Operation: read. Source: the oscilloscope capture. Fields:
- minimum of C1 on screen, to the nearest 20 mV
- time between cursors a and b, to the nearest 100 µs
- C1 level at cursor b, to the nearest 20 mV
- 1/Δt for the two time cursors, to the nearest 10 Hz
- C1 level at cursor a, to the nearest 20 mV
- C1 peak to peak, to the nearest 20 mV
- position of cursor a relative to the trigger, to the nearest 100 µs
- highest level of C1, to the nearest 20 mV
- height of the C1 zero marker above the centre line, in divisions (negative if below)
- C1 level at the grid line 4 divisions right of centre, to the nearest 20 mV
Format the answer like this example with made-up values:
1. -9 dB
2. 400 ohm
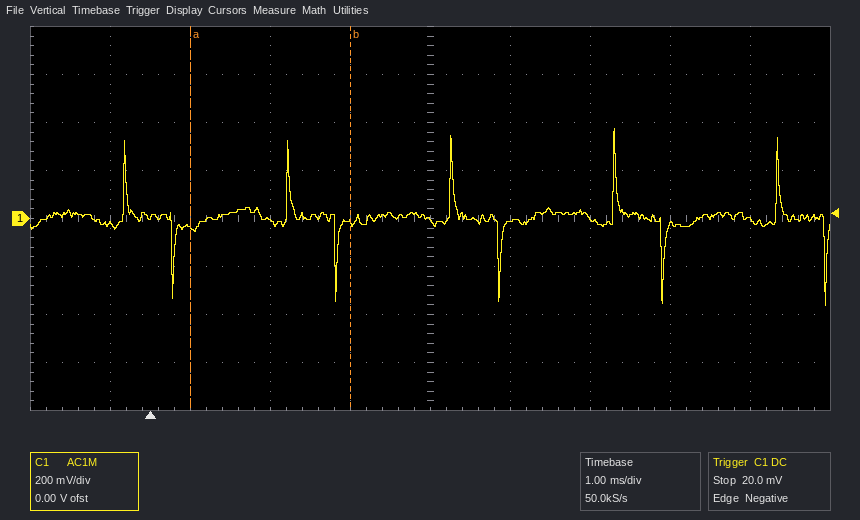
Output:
1. -360 mV
2. 2.0 ms
3. -20 mV
4. 500 Hz
5. -40 mV
6. 740 mV
7. +500 µs
8. 380 mV
9. 0.0 div
10. 0 mV
